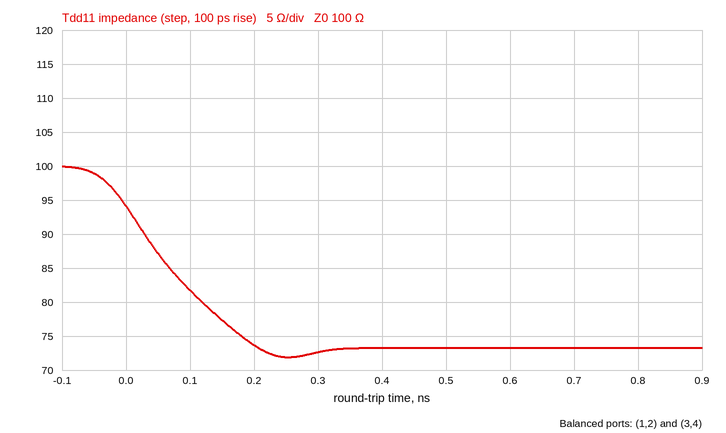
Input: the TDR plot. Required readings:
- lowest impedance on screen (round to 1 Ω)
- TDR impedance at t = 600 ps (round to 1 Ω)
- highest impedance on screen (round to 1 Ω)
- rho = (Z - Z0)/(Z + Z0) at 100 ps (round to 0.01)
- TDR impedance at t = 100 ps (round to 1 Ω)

72 Ω
73 Ω
100 Ω
-0.10
82 Ω
